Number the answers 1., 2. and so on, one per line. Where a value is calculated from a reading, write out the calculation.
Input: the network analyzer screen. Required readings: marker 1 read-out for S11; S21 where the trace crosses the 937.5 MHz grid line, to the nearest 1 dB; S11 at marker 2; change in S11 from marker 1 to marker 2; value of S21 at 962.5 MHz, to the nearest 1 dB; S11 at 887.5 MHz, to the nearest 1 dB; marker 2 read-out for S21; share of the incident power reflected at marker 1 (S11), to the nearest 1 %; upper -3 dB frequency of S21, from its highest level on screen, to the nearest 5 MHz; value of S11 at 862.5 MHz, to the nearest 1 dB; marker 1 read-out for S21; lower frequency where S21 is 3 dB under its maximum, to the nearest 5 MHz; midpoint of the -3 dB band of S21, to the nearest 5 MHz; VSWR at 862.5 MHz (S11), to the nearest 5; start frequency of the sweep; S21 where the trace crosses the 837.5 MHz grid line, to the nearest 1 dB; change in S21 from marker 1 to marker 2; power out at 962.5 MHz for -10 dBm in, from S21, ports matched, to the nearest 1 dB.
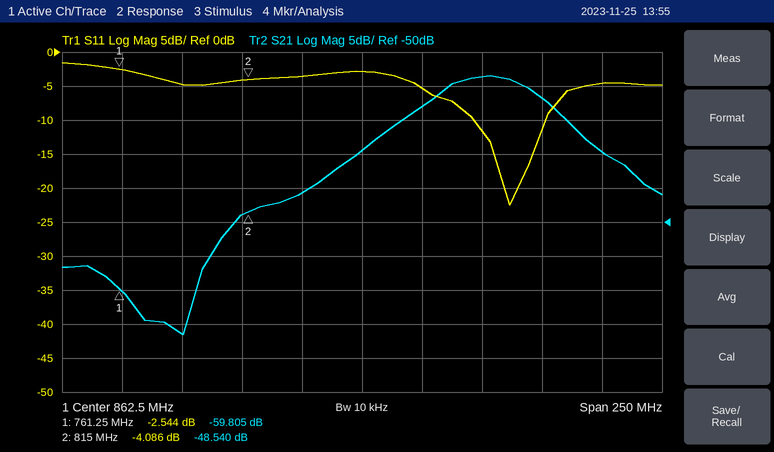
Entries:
1. -2.544 dB
2. -32 dB
3. -4.086 dB
4. -4.086 − (-2.544) = -1.542 dB
5. -40 dB
6. -5 dB
7. -48.540 dB
8. 10^(-2.544/10) ≈ 56 %
9. 935 MHz
10. -3 dB
11. -59.805 dB
12. 895 MHz
13. 915 MHz
14. |Γ| = 10^(-3/20) = 0.7079; VSWR = (1 + 0.7079)/(1 − 0.7079) ≈ 5.85, so 5 to the nearest 5
15. 737.5 MHz
16. -46 dB
17. -48.54 − (-59.805) = 11.265 dB
18. -10 dBm + (-40 dB) = -50 dBm
